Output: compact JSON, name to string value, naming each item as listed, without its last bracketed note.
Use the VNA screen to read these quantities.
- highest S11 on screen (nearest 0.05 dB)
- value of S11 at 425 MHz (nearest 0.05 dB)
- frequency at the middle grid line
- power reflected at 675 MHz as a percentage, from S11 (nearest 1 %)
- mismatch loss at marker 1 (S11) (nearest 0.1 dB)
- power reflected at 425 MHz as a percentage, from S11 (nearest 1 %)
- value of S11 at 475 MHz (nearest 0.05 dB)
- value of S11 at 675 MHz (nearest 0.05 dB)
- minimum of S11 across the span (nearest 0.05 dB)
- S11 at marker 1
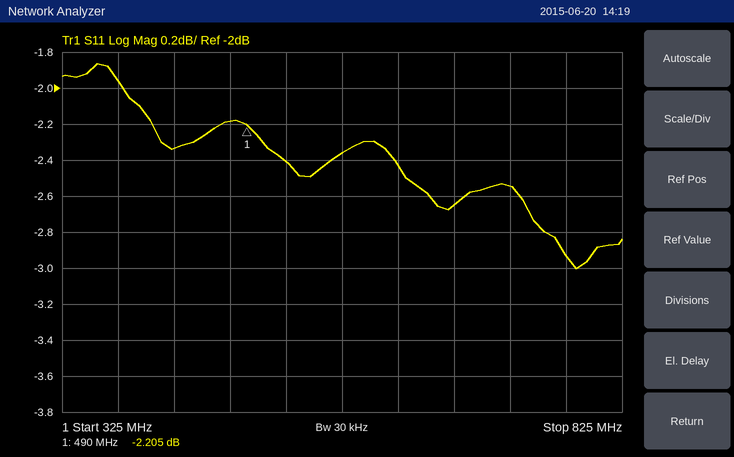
{"highest S11 on screen": "-1.85 dB", "value of S11 at 425 MHz": "-2.35 dB", "frequency at the middle grid line": "575 MHz", "power reflected at 675 MHz as a percentage, from S11": "54 %", "mismatch loss at marker 1 (S11)": "4.0 dB", "power reflected at 425 MHz as a percentage, from S11": "58 %", "value of S11 at 475 MHz": "-2.20 dB", "value of S11 at 675 MHz": "-2.65 dB", "minimum of S11 across the span": "-3.00 dB", "S11 at marker 1": "-2.205 dB"}
